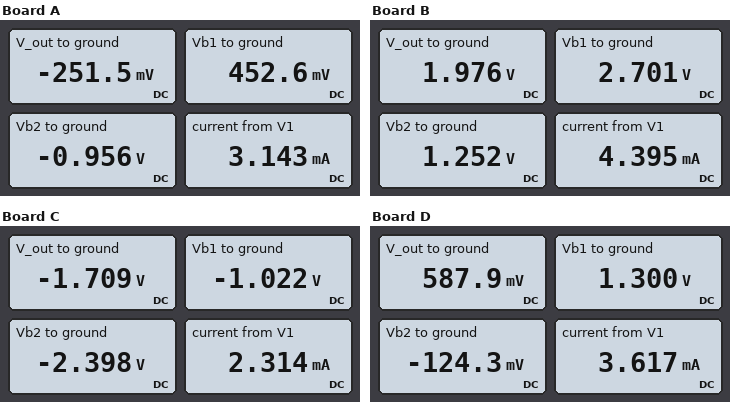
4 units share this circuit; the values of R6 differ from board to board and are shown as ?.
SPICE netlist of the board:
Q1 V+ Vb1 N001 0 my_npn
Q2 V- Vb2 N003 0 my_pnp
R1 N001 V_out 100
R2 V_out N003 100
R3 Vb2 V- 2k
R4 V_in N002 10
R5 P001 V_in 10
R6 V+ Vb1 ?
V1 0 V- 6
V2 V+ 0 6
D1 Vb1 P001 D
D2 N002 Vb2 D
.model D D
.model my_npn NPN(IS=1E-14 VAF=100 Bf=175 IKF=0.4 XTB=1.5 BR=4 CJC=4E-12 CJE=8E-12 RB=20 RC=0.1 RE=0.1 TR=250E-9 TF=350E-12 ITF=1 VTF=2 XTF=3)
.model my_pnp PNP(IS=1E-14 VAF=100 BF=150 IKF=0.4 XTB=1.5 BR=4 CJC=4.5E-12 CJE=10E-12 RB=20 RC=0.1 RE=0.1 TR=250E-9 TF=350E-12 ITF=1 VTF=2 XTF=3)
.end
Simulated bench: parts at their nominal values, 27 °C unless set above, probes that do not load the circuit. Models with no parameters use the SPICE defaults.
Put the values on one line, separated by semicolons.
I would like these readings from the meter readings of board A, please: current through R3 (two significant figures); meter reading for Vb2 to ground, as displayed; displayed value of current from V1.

2.5 mA; -0.956 V; 3.143 mA
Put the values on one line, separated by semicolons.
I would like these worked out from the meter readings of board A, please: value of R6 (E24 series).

2.2 kΩ
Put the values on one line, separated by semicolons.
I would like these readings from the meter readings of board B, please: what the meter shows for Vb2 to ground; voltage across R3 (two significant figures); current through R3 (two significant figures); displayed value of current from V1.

1.252 V; 7.3 V; 3.6 mA; 4.395 mA
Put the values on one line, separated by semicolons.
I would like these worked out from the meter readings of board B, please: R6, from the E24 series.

910 Ω
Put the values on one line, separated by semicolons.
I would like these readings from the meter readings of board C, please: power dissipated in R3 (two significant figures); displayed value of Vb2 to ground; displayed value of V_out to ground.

6.5 mW; -2.398 V; -1.709 V
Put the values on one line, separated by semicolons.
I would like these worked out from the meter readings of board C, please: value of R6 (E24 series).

3.9 kΩ
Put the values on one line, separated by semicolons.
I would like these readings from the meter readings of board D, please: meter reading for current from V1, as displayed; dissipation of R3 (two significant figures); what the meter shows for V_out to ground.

3.617 mA; 17 mW; 587.9 mV
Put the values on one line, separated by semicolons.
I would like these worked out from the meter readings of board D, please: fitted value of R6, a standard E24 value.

1.6 kΩ
